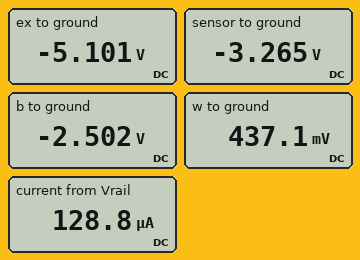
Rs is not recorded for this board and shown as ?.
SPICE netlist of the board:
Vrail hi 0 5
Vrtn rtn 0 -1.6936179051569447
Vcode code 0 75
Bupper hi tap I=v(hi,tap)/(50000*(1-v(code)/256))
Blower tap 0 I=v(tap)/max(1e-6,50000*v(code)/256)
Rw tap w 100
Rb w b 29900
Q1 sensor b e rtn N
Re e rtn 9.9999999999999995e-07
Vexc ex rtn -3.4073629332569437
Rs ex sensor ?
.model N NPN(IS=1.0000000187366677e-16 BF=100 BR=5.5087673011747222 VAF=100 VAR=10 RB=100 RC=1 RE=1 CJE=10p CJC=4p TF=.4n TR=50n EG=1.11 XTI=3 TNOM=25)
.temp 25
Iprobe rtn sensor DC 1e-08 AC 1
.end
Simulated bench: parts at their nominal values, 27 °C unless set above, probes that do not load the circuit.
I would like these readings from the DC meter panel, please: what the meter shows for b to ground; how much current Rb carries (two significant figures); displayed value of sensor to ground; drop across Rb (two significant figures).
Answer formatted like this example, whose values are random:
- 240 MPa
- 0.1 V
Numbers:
- -2.502 V
- 98 µA
- -3.265 V
- 2.9 V
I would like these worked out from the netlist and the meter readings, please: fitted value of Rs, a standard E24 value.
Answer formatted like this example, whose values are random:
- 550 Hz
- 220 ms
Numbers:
- 2.7 kΩ
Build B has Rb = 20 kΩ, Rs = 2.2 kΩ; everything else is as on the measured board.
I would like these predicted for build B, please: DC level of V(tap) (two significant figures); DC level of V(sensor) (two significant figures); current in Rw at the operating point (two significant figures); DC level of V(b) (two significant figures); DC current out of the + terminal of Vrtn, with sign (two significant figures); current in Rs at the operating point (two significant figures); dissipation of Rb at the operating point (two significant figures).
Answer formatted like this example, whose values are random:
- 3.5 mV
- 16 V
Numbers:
- 150 mV
- -3.2 V
- 130 µA
- -2.4 V
- -130 µA
- 870 µA
- 320 µW
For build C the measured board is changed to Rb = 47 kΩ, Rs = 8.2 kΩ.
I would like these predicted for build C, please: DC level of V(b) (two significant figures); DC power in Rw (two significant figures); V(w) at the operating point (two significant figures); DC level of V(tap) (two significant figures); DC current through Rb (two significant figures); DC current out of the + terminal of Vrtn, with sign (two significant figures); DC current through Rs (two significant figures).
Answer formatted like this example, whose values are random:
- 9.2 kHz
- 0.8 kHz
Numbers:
- -1.6 V
- 280 nW
- 910 mV
- 920 mV
- 53 µA
- -53 µA
- 340 µA
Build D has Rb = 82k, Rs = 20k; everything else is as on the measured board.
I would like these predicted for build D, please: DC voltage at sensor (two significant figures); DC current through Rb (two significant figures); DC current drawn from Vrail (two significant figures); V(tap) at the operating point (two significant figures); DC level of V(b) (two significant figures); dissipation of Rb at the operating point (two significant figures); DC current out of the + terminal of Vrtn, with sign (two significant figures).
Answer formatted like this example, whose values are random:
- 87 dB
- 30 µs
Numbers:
- -1.8 V
- 27 µA
- 110 µA
- 1.2 V
- -1.1 V
- 62 µW
- -27 µA
